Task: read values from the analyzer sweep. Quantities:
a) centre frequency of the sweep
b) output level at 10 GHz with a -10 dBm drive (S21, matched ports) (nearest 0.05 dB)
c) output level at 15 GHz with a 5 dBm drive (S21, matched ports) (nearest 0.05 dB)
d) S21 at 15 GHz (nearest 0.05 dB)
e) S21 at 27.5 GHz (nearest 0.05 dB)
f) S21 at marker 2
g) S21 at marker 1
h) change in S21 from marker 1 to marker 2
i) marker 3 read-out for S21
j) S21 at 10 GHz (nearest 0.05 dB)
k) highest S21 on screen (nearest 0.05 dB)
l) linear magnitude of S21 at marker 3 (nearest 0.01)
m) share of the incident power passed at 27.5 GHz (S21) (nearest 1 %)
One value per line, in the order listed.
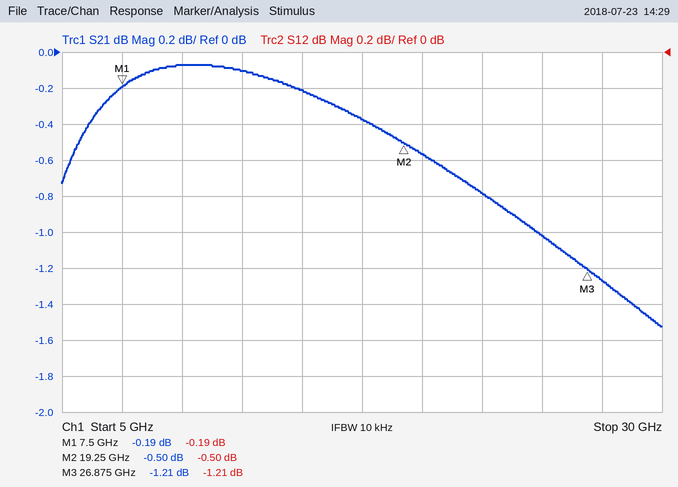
17.5 GHz
-10.05 dBm
4.80 dBm
-0.20 dB
-1.25 dB
-0.50 dB
-0.19 dB
-0.31 dB
-1.21 dB
-0.05 dB
-0.05 dB
0.87
75 %
